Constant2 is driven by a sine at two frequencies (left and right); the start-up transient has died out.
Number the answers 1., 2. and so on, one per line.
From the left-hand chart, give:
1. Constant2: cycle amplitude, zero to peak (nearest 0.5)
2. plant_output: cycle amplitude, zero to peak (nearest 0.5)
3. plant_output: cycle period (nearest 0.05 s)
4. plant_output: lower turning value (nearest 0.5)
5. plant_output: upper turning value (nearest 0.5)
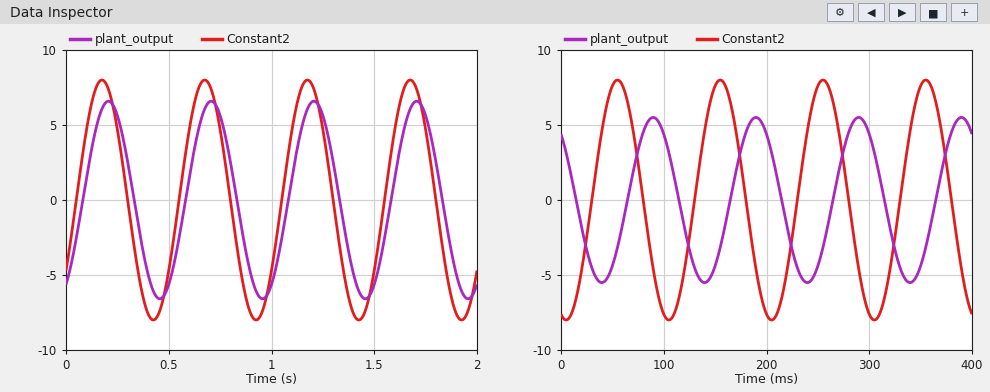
1. 8.0
2. 6.5
3. 0.50 s
4. -6.5
5. 6.5
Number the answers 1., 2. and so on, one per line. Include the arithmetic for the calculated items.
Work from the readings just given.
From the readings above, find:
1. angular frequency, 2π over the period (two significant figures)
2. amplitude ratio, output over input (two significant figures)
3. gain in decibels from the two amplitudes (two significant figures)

1. 2π / 0.5 = 13 rad/s
2. 6.5 / 8 = 0.81
3. 20 log10(6.5 / 8) = -1.8 dB
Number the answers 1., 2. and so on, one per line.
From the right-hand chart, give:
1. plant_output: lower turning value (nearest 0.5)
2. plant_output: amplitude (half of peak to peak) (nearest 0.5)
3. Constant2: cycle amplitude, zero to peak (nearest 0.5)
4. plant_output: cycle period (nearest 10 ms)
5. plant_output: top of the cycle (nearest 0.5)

1. -5.5
2. 5.5
3. 8.0
4. 100 ms
5. 5.5
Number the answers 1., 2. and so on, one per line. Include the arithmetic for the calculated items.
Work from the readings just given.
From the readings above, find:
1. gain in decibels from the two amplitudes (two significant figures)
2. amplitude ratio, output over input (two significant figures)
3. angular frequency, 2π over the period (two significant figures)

1. 20 log10(5.5 / 8) = -3.3 dB
2. 5.5 / 8 = 0.69
3. 2π / 100 = 0.063 rad/ms
